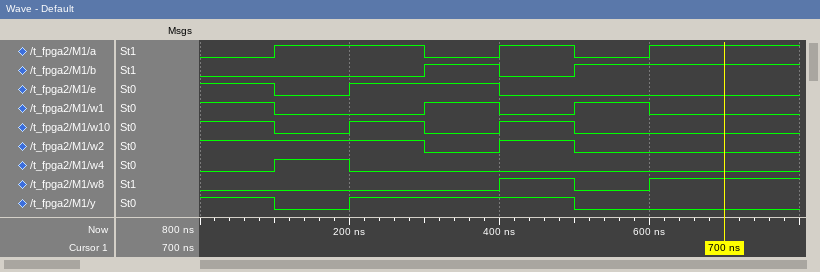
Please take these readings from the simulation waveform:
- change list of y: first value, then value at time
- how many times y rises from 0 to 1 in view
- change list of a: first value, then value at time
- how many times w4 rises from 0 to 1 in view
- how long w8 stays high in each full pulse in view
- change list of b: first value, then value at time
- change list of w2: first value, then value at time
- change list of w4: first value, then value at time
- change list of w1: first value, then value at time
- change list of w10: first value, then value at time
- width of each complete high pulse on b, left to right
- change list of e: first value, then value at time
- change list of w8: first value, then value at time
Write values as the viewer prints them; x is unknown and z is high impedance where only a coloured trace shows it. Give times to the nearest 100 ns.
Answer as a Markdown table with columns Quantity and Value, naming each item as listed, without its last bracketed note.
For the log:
| Quantity | Value |
|---|---|
| change list of y: first value, then value at time | 1, 0 at 100 ns, 1 at 200 ns, 0 at 500 ns |
| how many times y rises from 0 to 1 in view | 1 |
| change list of a: first value, then value at time | 0, 1 at 100 ns, 0 at 300 ns, 1 at 400 ns, 0 at 500 ns, 1 at 600 ns |
| how many times w4 rises from 0 to 1 in view | 1 |
| how long w8 stays high in each full pulse in view | 100 ns |
| change list of b: first value, then value at time | 0, 1 at 300 ns, 0 at 400 ns, 1 at 500 ns |
| change list of w2: first value, then value at time | 1, 0 at 300 ns, 1 at 400 ns, 0 at 500 ns |
| change list of w4: first value, then value at time | 0, 1 at 100 ns, 0 at 200 ns |
| change list of w1: first value, then value at time | 1, 0 at 100 ns, 1 at 300 ns, 0 at 400 ns, 1 at 500 ns, 0 at 600 ns |
| change list of w10: first value, then value at time | 1, 0 at 100 ns, 1 at 200 ns, 0 at 300 ns, 1 at 400 ns, 0 at 500 ns |
| width of each complete high pulse on b, left to right | 100 ns |
| change list of e: first value, then value at time | 1, 0 at 100 ns, 1 at 200 ns, 0 at 400 ns |
| change list of w8: first value, then value at time | 0, 1 at 400 ns, 0 at 500 ns, 1 at 600 ns |
